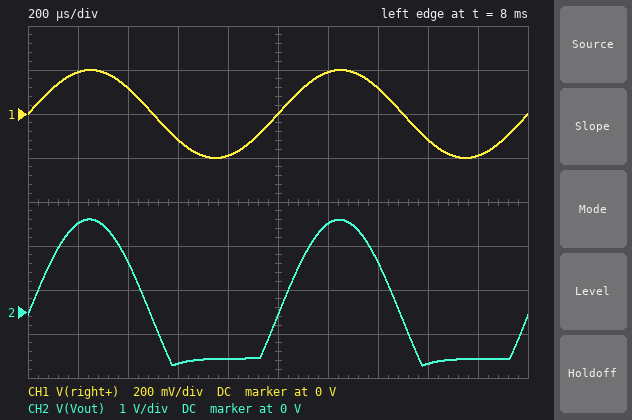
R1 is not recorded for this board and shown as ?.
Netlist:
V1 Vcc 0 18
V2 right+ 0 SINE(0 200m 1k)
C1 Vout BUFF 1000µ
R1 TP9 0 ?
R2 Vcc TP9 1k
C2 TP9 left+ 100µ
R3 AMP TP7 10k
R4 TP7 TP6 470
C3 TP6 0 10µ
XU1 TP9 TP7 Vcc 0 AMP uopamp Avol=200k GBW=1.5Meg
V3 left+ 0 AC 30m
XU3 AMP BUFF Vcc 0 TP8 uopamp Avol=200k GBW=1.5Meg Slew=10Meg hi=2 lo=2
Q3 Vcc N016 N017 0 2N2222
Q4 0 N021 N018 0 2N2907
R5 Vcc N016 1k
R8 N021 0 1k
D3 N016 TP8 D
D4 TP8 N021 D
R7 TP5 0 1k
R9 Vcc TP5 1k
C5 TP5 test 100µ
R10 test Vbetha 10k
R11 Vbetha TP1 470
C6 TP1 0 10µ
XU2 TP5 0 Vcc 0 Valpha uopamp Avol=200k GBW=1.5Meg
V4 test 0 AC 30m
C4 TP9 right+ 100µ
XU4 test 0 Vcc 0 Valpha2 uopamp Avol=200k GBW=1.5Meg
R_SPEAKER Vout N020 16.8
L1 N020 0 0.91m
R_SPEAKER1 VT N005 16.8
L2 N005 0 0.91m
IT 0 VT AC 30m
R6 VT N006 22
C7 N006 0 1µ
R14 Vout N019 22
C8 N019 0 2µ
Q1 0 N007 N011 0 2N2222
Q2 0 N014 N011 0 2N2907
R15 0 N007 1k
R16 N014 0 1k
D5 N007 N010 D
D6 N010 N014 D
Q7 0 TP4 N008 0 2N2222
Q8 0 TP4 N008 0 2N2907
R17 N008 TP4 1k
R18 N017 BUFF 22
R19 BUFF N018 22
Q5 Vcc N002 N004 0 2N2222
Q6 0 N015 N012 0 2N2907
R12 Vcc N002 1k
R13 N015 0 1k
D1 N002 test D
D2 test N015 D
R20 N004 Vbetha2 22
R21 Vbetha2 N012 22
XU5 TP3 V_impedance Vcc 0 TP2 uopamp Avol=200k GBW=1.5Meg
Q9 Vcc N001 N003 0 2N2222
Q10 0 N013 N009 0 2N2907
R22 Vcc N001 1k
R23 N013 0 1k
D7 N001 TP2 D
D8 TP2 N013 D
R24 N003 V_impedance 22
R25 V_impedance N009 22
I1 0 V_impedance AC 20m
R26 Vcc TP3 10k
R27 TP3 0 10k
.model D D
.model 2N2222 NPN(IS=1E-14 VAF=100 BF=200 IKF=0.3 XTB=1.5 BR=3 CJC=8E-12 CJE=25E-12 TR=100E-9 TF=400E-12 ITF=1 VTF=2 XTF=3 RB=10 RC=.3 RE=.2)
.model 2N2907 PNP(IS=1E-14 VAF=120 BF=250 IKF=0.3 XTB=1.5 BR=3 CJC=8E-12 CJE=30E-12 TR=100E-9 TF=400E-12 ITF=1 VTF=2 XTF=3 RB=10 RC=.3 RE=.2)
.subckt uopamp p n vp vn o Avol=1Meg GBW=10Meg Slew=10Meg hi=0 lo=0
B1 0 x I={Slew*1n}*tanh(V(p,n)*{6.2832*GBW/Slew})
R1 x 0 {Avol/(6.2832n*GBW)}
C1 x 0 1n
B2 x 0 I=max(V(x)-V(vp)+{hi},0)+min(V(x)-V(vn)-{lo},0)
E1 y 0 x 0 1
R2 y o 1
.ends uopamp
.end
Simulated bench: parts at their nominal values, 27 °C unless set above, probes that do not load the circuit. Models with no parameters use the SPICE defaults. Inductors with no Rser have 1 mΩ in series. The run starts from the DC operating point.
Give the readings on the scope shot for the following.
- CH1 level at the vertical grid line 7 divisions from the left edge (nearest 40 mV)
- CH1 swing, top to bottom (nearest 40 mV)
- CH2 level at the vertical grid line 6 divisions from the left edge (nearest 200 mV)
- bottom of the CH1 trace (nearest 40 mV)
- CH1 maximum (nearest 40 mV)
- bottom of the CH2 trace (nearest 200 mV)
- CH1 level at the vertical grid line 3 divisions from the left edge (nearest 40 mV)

120 mV
400 mV
2.0 V
-200 mV
200 mV
-1.2 V
-120 mV
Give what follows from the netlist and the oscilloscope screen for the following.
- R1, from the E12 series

330 Ω
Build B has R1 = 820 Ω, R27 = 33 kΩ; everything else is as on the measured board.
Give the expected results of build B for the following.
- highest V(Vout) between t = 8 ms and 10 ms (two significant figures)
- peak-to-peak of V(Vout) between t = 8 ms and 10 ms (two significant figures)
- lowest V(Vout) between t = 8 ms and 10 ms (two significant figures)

2.2 V
4.5 V
-2.2 V
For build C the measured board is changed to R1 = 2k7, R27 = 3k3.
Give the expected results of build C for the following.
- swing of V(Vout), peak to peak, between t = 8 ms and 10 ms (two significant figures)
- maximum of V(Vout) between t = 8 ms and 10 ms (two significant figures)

3.5 V
1.4 V
